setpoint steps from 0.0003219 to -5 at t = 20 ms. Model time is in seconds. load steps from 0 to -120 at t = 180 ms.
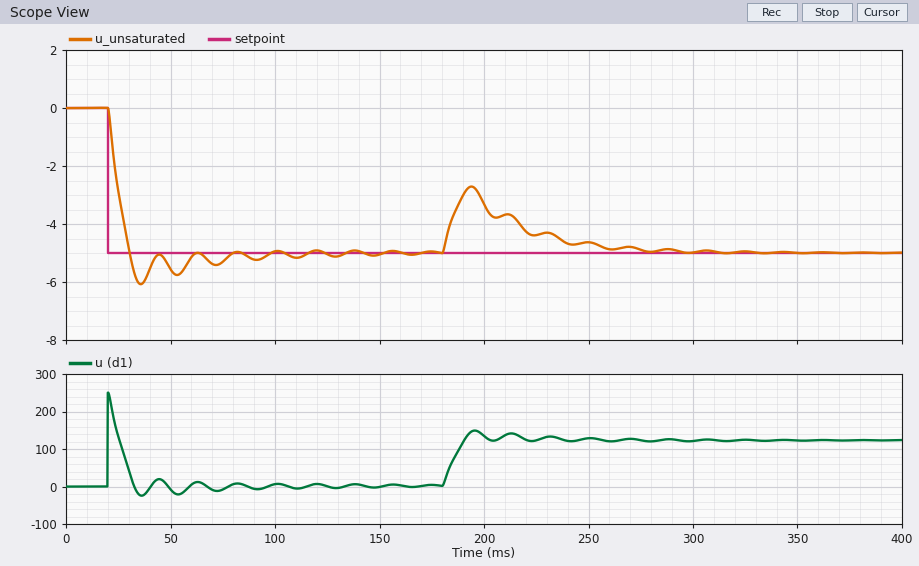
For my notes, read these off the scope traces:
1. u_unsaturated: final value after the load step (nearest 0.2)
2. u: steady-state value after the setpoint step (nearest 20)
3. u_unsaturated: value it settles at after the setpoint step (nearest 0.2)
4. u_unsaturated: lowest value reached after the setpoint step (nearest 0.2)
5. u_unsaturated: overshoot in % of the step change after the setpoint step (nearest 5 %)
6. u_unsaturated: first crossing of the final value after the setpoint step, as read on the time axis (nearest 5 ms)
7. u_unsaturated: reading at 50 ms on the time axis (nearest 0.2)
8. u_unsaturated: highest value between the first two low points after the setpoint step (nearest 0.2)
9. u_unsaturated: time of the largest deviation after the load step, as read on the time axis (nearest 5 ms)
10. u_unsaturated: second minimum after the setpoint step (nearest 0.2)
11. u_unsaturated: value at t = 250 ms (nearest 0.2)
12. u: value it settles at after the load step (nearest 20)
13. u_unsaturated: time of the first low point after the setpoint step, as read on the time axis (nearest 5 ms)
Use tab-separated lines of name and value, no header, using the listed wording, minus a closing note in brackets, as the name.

u_unsaturated: final value after the load step	-5.0
u: steady-state value after the setpoint step	0
u_unsaturated: value it settles at after the setpoint step	-5.0
u_unsaturated: lowest value reached after the setpoint step	-6.0
u_unsaturated: overshoot in % of the step change after the setpoint step	20 %
u_unsaturated: first crossing of the final value after the setpoint step, as read on the time axis	30 ms
u_unsaturated: reading at 50 ms on the time axis	-5.6
u_unsaturated: highest value between the first two low points after the setpoint step	-5.0
u_unsaturated: time of the largest deviation after the load step, as read on the time axis	195 ms
u_unsaturated: second minimum after the setpoint step	-5.8
u_unsaturated: value at t = 250 ms	-4.6
u: value it settles at after the load step	120
u_unsaturated: time of the first low point after the setpoint step, as read on the time axis	35 ms
